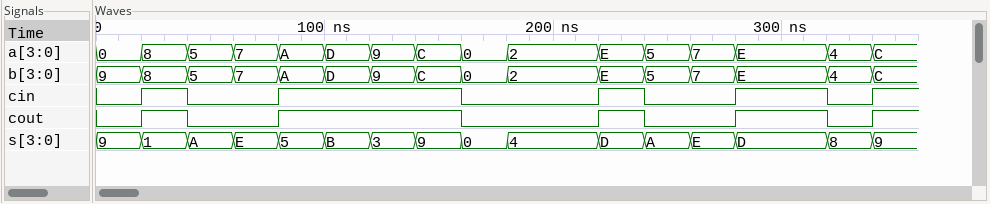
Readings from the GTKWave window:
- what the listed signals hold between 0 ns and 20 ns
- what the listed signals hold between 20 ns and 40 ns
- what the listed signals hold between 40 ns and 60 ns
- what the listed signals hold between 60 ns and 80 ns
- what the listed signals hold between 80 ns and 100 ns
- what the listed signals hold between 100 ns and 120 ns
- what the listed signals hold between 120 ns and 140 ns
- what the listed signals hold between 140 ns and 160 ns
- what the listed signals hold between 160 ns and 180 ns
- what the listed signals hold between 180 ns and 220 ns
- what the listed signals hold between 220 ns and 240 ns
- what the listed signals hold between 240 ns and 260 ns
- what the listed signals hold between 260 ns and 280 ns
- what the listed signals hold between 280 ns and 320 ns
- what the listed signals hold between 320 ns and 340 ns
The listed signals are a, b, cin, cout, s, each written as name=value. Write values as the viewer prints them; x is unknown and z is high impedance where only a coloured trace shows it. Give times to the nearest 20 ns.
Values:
a=0, b=9, cin=0, cout=0, s=9
a=8, b=8, cin=1, cout=1, s=1
a=5, b=5, cin=0, cout=0, s=A
a=7, b=7, cin=0, cout=0, s=E
a=A, b=A, cin=1, cout=1, s=5
a=D, b=D, cin=1, cout=1, s=B
a=9, b=9, cin=1, cout=1, s=3
a=C, b=C, cin=1, cout=1, s=9
a=0, b=0, cin=0, cout=0, s=0
a=2, b=2, cin=0, cout=0, s=4
a=E, b=E, cin=1, cout=1, s=D
a=5, b=5, cin=0, cout=0, s=A
a=7, b=7, cin=0, cout=0, s=E
a=E, b=E, cin=1, cout=1, s=D
a=4, b=4, cin=0, cout=0, s=8
